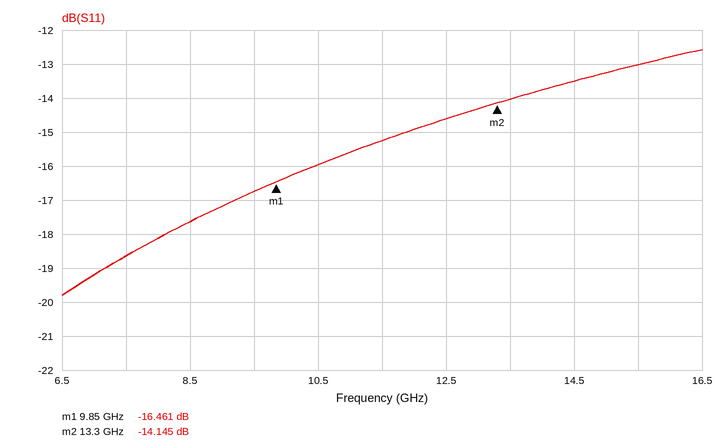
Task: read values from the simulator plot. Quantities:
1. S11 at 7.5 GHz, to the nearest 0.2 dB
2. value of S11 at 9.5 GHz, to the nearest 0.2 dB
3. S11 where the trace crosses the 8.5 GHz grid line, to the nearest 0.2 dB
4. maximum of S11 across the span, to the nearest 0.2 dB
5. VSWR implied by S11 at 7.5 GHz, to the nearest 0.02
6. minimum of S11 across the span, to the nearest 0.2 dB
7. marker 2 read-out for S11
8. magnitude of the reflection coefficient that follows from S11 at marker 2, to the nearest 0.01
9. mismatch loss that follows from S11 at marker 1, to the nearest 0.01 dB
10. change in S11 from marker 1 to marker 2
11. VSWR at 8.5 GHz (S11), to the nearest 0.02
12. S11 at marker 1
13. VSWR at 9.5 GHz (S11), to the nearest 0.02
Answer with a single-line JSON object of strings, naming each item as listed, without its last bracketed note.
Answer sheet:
{"S11 at 7.5 GHz, to the nearest 0.2 dB": "-18.6 dB", "value of S11 at 9.5 GHz, to the nearest 0.2 dB": "-16.8 dB", "S11 where the trace crosses the 8.5 GHz grid line, to the nearest 0.2 dB": "-17.6 dB", "maximum of S11 across the span, to the nearest 0.2 dB": "-12.6 dB", "VSWR implied by S11 at 7.5 GHz, to the nearest 0.02": "1.26", "minimum of S11 across the span, to the nearest 0.2 dB": "-19.8 dB", "marker 2 read-out for S11": "-14.145 dB", "magnitude of the reflection coefficient that follows from S11 at marker 2, to the nearest 0.01": "0.20", "mismatch loss that follows from S11 at marker 1, to the nearest 0.01 dB": "0.10 dB", "change in S11 from marker 1 to marker 2": "2.316 dB", "VSWR at 8.5 GHz (S11), to the nearest 0.02": "1.30", "S11 at marker 1": "-16.461 dB", "VSWR at 9.5 GHz (S11), to the nearest 0.02": "1.34"}
